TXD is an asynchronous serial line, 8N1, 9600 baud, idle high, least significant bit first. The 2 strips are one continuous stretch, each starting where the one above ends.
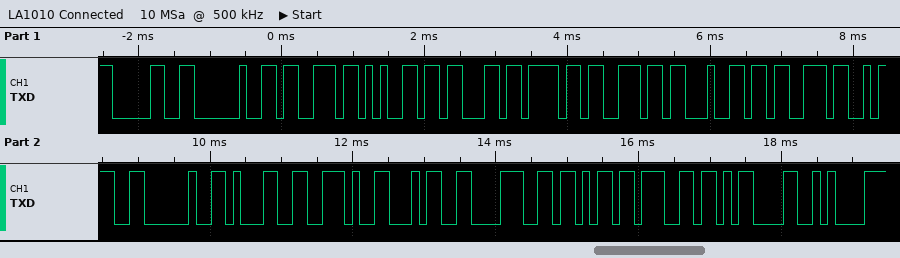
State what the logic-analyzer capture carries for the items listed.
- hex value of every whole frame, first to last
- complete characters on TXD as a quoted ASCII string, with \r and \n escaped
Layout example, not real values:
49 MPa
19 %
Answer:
30 20 73 65 63 6F 6E 64 73 3A 20 31 2E 34 38 6B 67 0D 0A
"0 seconds: 1.48kg\r\n"
